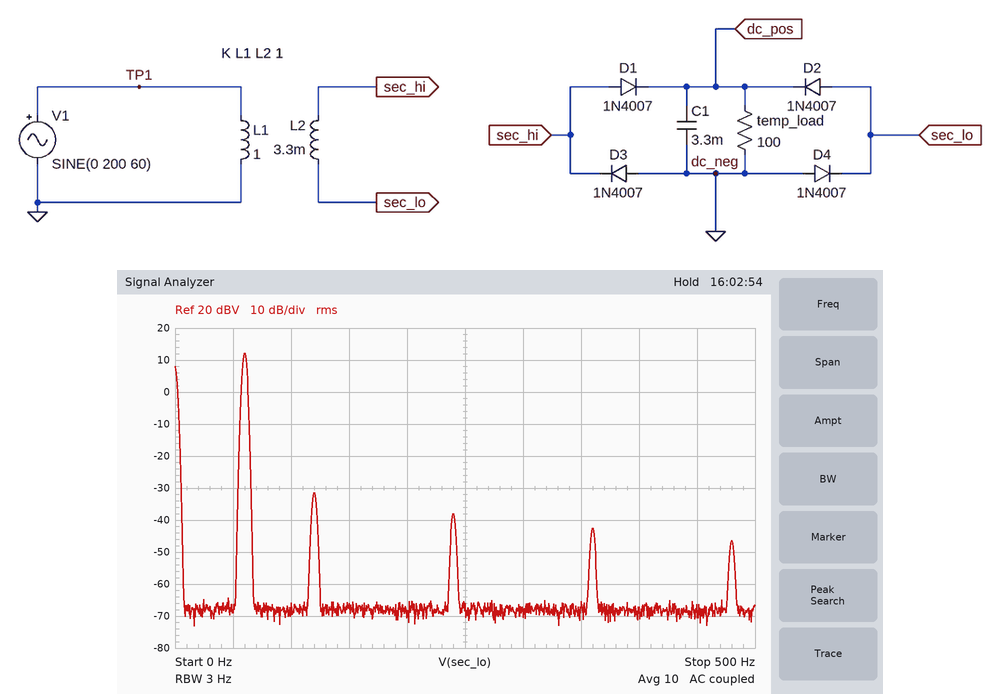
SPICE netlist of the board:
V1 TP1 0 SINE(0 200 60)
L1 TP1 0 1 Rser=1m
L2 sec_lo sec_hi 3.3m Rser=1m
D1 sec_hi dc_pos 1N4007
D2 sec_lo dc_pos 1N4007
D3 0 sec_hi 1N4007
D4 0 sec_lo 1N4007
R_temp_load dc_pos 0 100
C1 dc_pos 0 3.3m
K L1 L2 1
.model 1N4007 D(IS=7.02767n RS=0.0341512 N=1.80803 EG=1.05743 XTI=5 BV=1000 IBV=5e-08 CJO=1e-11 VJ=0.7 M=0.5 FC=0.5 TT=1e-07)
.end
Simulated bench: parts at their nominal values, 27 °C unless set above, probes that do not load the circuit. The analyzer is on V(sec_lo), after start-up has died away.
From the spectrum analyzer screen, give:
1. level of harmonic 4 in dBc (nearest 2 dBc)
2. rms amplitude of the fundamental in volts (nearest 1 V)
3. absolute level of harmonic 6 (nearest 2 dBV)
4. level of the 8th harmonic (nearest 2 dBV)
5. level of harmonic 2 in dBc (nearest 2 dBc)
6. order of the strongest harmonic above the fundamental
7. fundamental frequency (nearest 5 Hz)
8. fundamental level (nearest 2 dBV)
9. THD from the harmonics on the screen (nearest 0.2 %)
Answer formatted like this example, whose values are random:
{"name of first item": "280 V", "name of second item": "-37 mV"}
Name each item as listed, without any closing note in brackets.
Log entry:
{"level of harmonic 4 in dBc": "-50 dBc", "rms amplitude of the fundamental in volts": "4 V", "absolute level of harmonic 6": "-42 dBV", "level of the 8th harmonic": "-46 dBV", "level of harmonic 2 in dBc": "-44 dBc", "order of the strongest harmonic above the fundamental": "2", "fundamental frequency": "60 Hz", "fundamental level": "12 dBV", "THD from the harmonics on the screen": "0.8 %"}
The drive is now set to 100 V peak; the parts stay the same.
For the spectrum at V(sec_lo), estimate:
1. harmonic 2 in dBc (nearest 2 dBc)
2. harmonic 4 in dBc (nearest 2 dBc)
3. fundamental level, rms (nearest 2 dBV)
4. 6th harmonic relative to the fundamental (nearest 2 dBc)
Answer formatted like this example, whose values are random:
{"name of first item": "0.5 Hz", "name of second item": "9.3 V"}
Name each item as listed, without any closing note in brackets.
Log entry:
{"harmonic 2 in dBc": "-46 dBc", "harmonic 4 in dBc": "-52 dBc", "fundamental level, rms": "6 dBV", "6th harmonic relative to the fundamental": "-58 dBc"}
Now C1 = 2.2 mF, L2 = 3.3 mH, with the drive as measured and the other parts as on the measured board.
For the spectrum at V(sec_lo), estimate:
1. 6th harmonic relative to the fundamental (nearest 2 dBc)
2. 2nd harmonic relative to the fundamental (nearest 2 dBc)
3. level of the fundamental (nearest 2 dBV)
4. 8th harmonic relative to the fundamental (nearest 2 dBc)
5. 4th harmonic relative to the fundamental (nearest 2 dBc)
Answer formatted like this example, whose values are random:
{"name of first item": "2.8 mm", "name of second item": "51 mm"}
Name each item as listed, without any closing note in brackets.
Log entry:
{"6th harmonic relative to the fundamental": "-52 dBc", "2nd harmonic relative to the fundamental": "-40 dBc", "level of the fundamental": "12 dBV", "8th harmonic relative to the fundamental": "-56 dBc", "4th harmonic relative to the fundamental": "-46 dBc"}
